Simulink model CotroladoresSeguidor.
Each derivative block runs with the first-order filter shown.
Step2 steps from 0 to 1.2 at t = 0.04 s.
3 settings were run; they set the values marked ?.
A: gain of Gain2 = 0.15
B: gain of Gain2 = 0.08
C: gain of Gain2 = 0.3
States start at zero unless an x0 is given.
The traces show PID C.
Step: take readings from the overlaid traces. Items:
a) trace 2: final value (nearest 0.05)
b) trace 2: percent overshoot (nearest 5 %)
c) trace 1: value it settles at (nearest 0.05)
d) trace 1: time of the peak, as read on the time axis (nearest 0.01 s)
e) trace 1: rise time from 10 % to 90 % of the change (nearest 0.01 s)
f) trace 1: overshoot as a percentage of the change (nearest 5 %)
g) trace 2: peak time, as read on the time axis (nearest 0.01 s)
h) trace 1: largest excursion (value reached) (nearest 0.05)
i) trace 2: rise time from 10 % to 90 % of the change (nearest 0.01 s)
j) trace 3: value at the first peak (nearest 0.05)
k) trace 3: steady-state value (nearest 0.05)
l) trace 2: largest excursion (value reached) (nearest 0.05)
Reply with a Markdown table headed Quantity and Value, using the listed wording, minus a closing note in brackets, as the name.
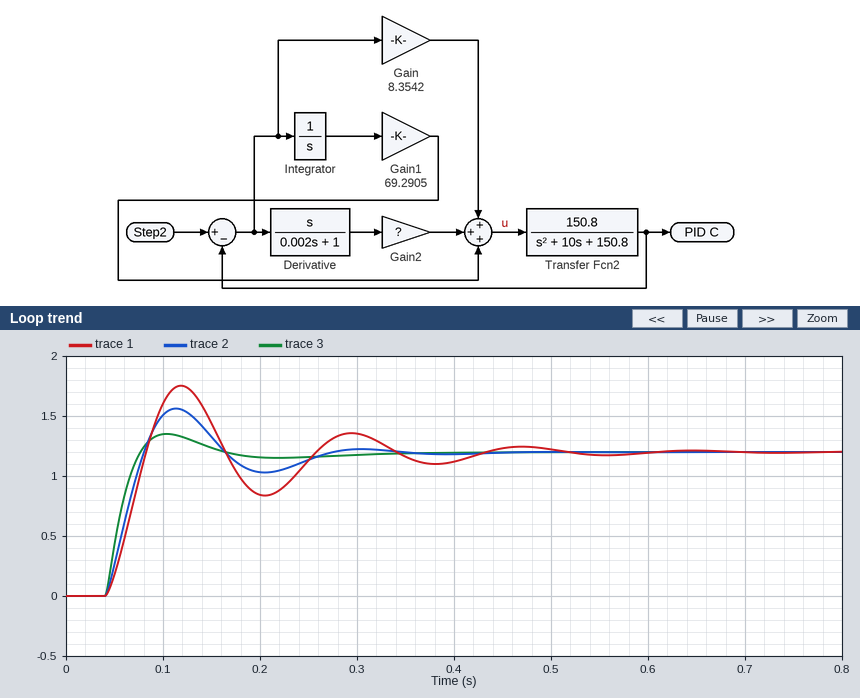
| Quantity | Value |
|---|---|
| trace 2: final value | 1.20 |
| trace 2: percent overshoot | 30 % |
| trace 1: value it settles at | 1.20 |
| trace 1: time of the peak, as read on the time axis | 0.12 s |
| trace 1: rise time from 10 % to 90 % of the change | 0.03 s |
| trace 1: overshoot as a percentage of the change | 45 % |
| trace 2: peak time, as read on the time axis | 0.11 s |
| trace 1: largest excursion (value reached) | 1.75 |
| trace 2: rise time from 10 % to 90 % of the change | 0.03 s |
| trace 3: value at the first peak | 1.35 |
| trace 3: steady-state value | 1.20 |
| trace 2: largest excursion (value reached) | 1.55 |
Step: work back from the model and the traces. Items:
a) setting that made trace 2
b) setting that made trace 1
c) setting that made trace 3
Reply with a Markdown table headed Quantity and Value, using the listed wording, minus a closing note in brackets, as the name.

| Quantity | Value |
|---|---|
| setting that made trace 2 | A |
| setting that made trace 1 | B |
| setting that made trace 3 | C |
